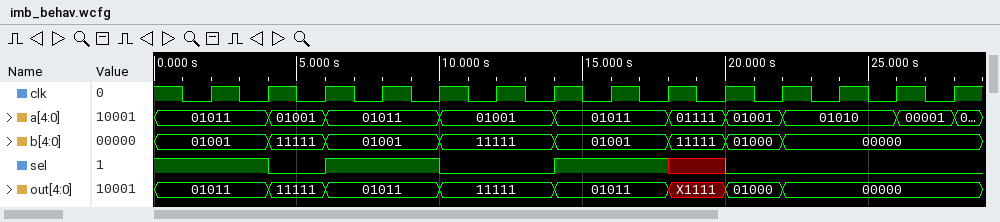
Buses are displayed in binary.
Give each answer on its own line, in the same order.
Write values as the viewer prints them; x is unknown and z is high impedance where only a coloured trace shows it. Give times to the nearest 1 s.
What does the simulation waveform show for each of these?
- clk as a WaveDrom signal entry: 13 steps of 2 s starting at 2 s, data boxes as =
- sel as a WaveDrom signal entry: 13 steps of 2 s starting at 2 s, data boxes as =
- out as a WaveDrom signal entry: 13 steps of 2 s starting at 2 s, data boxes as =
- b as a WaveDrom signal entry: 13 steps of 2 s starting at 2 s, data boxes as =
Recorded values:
{name: 'clk', wave: 'p............'}
{name: 'sel', wave: '101.0.1.x0...'}
{name: 'out', wave: '===.=.=.===..', data: '01011 11111 01011 11111 01011 X1111 01000 00000'}
{name: 'b', wave: '===.=.=.===..', data: '01001 11111 01001 11111 01001 11111 01000 00000'}
